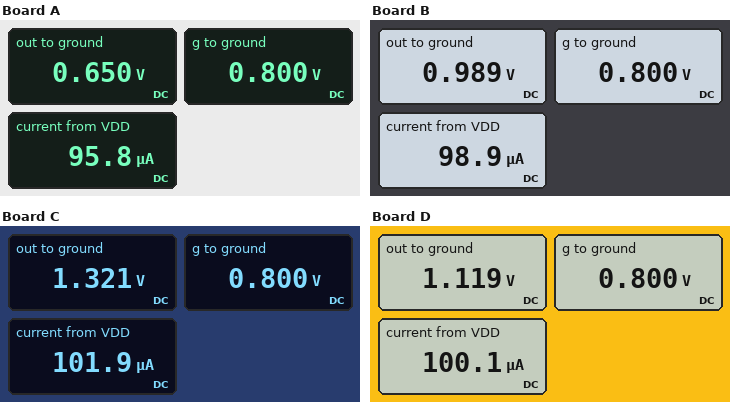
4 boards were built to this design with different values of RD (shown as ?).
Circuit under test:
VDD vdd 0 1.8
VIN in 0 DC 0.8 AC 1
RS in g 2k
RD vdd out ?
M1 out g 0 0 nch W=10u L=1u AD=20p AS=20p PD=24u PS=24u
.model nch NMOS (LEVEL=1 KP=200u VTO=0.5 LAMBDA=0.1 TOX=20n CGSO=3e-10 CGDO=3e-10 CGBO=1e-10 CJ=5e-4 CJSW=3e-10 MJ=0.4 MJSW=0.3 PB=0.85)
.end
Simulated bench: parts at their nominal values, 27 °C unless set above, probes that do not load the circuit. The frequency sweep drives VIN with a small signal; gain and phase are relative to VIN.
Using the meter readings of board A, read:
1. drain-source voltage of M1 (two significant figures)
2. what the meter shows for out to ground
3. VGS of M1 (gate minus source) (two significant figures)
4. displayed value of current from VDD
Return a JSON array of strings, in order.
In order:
["650 mV", "0.650 V", "800 mV", "95.8 µA"]
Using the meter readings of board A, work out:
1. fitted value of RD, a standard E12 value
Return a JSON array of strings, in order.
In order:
["12 kΩ"]
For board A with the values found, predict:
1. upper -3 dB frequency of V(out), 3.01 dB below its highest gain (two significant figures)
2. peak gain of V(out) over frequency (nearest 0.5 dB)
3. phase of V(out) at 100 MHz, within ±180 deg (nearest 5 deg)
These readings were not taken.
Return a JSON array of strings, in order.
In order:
["670 MHz", "17.0 dB", "170 deg"]
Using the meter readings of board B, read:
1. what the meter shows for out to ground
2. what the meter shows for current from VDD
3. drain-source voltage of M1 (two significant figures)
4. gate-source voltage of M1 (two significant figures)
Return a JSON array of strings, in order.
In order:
["0.989 V", "98.9 µA", "990 mV", "800 mV"]
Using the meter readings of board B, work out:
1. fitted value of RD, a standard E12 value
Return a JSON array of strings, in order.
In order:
["8.2 kΩ"]
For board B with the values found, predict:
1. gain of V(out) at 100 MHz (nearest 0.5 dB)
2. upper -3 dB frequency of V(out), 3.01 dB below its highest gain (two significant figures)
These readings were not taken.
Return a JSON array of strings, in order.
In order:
["14.0 dB", "960 MHz"]
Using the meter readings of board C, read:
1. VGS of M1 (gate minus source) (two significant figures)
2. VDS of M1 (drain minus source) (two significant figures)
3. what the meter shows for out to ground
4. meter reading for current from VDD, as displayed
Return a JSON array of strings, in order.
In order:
["800 mV", "1.3 V", "1.321 V", "101.9 µA"]
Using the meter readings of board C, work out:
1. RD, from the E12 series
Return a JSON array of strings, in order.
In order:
["4.7 kΩ"]
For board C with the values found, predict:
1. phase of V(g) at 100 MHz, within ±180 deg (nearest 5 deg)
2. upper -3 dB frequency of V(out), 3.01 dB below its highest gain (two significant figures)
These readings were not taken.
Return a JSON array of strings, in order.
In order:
["0 deg", "1.5 GHz"]
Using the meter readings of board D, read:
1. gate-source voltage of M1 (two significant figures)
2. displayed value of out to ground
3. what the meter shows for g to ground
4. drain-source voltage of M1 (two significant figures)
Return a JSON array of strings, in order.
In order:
["800 mV", "1.119 V", "0.800 V", "1.1 V"]
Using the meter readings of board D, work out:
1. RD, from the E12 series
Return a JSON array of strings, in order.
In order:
["6.8 kΩ"]
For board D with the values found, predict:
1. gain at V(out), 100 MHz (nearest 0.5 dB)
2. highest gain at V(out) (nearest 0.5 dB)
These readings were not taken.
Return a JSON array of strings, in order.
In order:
["12.5 dB", "12.5 dB"]
